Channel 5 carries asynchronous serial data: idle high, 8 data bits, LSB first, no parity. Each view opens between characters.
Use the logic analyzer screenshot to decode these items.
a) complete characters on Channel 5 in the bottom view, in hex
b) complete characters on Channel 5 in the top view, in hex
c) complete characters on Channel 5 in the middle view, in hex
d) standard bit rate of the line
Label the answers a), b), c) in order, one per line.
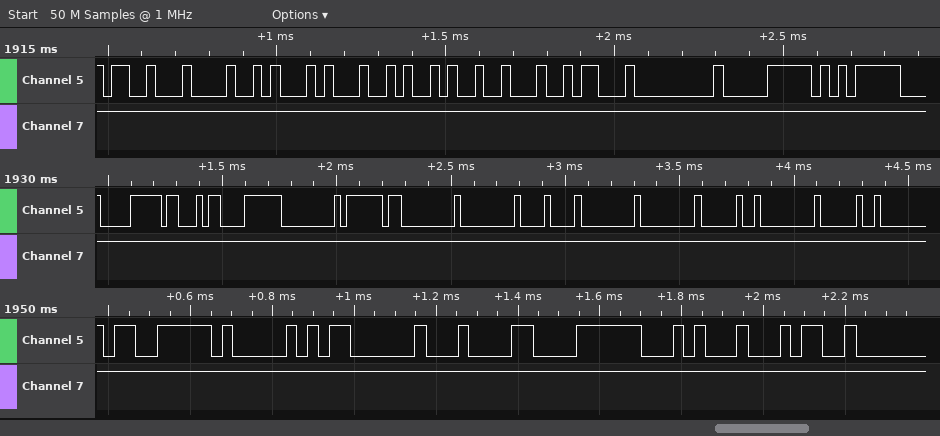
a) F3, 41, 03, 84, F8, 14, 34
b) 13, 48, 14, 4A, 12, 1A, 00, F0, F5
c) F0, A3, F8, 00, BF, 00, 00, 08, 00, 00, 20, 00, 20
d) 38400 baud
